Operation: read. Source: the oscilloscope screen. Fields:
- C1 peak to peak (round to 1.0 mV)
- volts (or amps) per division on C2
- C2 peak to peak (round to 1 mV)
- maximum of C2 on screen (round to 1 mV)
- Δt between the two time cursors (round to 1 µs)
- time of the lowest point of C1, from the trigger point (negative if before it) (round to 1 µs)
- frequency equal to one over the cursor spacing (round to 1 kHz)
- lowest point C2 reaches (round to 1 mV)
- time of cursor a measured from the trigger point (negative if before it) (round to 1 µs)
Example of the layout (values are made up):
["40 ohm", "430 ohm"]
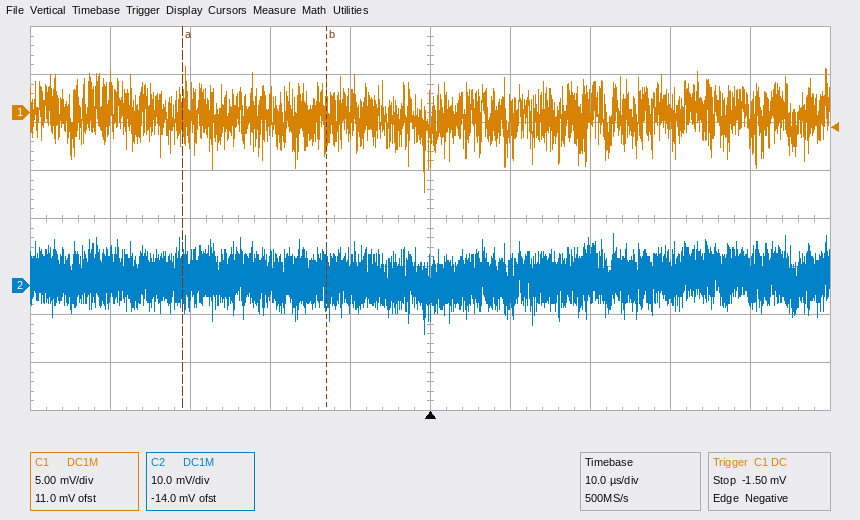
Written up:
["13.0 mV", "10 mV", "21 mV", "11 mV", "18 µs", "-1 µs", "56 kHz", "-10 mV", "-31 µs"]
